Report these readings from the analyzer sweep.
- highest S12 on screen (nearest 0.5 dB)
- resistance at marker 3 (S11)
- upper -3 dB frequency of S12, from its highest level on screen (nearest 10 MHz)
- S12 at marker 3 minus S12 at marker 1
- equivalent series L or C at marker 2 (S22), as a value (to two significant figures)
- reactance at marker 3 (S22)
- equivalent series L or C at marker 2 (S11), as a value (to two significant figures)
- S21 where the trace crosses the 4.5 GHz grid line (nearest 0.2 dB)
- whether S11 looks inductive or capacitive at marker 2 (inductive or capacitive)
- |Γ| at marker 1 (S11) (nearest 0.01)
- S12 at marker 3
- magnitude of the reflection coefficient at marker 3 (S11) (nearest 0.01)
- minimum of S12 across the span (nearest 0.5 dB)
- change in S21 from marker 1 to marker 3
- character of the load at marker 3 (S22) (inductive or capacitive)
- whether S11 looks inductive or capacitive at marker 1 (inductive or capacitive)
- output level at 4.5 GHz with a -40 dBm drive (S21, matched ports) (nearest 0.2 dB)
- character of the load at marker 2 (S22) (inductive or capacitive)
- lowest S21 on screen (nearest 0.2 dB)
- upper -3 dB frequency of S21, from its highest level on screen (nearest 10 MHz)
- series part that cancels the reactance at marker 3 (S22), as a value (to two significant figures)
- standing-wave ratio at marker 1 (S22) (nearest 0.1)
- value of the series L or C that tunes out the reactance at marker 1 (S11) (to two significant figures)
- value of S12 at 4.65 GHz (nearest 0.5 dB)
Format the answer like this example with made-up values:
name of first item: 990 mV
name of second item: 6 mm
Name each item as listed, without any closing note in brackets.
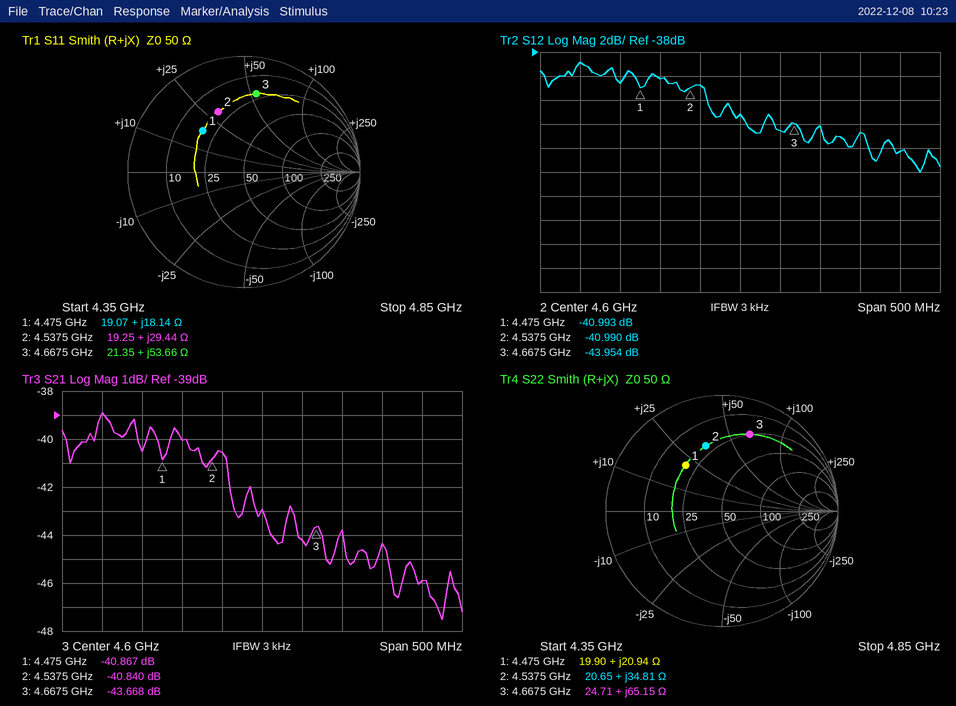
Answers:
highest S12 on screen: -39.0 dB
resistance at marker 3: 21.35 Ω
upper -3 dB frequency of S12, from its highest level on screen: 4.56 GHz
S12 at marker 3 minus S12 at marker 1: -2.961 dB
equivalent series L or C at marker 2 (S22), as a value: 1.2 nH
reactance at marker 3: +65.15 Ω
equivalent series L or C at marker 2 (S11), as a value: 1.0 nH
S21 where the trace crosses the 4.5 GHz grid line: -40.0 dB
whether S11 looks inductive or capacitive at marker 2: inductive
|Γ| at marker 1 (S11): 0.50
S12 at marker 3: -43.954 dB
magnitude of the reflection coefficient at marker 3 (S11): 0.68
minimum of S12 across the span: -48.0 dB
change in S21 from marker 1 to marker 3: -2.801 dB
character of the load at marker 3 (S22): inductive
whether S11 looks inductive or capacitive at marker 1: inductive
output level at 4.5 GHz with a -40 dBm drive (S21, matched ports): -80.0 dBm
character of the load at marker 2 (S22): inductive
lowest S21 on screen: -47.6 dB
upper -3 dB frequency of S21, from its highest level on screen: 4.56 GHz
series part that cancels the reactance at marker 3 (S22), as a value: 520 fF
standing-wave ratio at marker 1 (S22): 3.0
value of the series L or C that tunes out the reactance at marker 1 (S11): 2.0 pF
value of S12 at 4.65 GHz: -44.5 dB
